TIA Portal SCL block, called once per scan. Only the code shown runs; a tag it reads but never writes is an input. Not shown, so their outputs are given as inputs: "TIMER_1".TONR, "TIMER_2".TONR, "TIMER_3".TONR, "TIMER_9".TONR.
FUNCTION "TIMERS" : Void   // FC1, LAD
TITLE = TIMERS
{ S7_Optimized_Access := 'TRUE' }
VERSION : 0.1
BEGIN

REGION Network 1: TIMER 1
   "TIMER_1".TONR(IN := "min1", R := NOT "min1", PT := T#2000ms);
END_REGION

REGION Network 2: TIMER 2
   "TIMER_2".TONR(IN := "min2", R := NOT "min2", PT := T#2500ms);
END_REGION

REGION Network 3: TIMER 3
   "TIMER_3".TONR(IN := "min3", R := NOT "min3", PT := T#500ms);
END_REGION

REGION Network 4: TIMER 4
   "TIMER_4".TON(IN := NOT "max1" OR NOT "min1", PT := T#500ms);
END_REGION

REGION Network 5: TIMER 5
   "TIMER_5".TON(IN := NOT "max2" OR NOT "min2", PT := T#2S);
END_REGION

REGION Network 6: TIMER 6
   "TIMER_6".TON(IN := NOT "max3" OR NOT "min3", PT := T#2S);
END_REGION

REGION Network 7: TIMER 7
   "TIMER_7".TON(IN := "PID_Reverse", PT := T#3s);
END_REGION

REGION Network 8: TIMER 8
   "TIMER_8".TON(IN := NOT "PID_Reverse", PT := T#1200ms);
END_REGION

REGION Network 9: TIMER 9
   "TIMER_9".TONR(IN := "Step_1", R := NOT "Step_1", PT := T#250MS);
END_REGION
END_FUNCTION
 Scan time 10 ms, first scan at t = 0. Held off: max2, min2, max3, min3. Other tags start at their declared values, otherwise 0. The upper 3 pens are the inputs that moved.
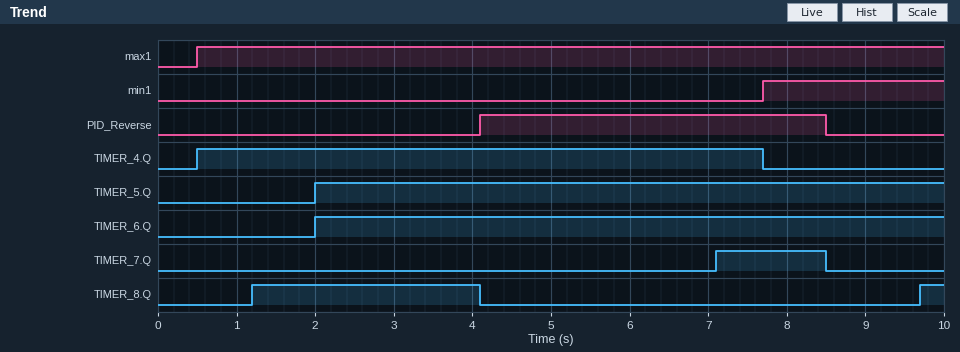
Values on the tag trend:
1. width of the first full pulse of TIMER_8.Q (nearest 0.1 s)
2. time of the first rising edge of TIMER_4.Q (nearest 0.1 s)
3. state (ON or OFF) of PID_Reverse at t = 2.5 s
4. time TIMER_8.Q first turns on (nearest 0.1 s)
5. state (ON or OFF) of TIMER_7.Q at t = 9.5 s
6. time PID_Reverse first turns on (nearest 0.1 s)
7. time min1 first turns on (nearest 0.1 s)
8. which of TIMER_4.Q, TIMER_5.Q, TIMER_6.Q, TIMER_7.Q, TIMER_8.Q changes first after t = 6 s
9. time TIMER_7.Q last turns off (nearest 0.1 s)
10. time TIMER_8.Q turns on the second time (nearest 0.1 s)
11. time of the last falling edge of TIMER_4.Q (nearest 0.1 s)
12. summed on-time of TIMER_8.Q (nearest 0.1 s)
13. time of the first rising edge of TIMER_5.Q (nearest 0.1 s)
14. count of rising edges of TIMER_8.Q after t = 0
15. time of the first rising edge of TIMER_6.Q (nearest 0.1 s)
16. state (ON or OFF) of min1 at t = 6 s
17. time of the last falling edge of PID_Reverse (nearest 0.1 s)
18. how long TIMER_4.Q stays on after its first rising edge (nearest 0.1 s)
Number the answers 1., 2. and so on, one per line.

1. 2.9 s
2. 0.5 s
3. OFF
4. 1.2 s
5. OFF
6. 4.1 s
7. 7.7 s
8. TIMER_7.Q
9. 8.5 s
10. 9.7 s
11. 7.7 s
12. 3.2 s
13. 2.0 s
14. 2
15. 2.0 s
16. OFF
17. 8.5 s
18. 7.2 s
